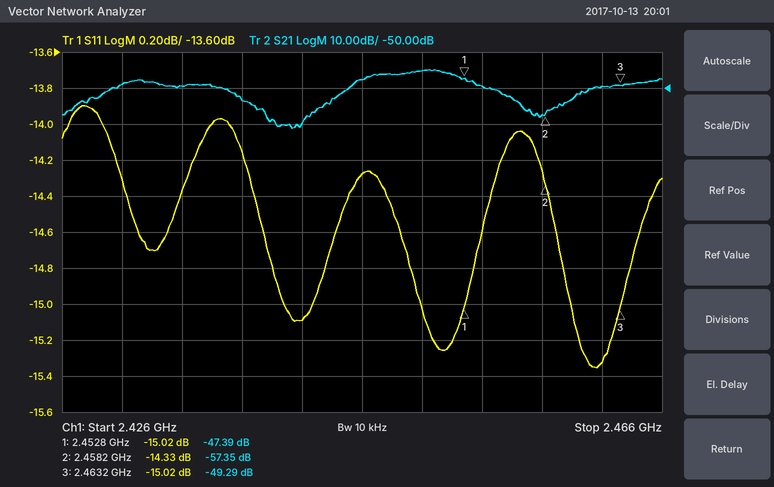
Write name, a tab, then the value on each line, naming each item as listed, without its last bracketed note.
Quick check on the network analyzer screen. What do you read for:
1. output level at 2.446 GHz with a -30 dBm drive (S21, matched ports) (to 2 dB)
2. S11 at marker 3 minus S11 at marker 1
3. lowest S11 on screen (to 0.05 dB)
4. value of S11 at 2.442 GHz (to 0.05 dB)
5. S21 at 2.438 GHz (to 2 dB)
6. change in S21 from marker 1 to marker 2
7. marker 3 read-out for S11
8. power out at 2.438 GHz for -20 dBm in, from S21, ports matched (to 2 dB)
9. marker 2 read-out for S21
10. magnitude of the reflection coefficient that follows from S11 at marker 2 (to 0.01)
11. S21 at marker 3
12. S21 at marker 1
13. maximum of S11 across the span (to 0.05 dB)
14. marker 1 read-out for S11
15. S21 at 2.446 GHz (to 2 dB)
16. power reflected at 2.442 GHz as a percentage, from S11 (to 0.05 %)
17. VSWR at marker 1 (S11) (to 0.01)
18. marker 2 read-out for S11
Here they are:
output level at 2.446 GHz with a -30 dBm drive (S21, matched ports)	-78 dBm
S11 at marker 3 minus S11 at marker 1	0.00 dB
lowest S11 on screen	-15.35 dB
value of S11 at 2.442 GHz	-15.10 dB
S21 at 2.438 GHz	-54 dB
change in S21 from marker 1 to marker 2	-9.96 dB
marker 3 read-out for S11	-15.02 dB
power out at 2.438 GHz for -20 dBm in, from S21, ports matched	-74 dBm
marker 2 read-out for S21	-57.35 dB
magnitude of the reflection coefficient that follows from S11 at marker 2	0.19
S21 at marker 3	-49.29 dB
S21 at marker 1	-47.39 dB
maximum of S11 across the span	-13.90 dB
marker 1 read-out for S11	-15.02 dB
S21 at 2.446 GHz	-48 dB
power reflected at 2.442 GHz as a percentage, from S11	3.10 %
VSWR at marker 1 (S11)	1.43
marker 2 read-out for S11	-14.33 dB
